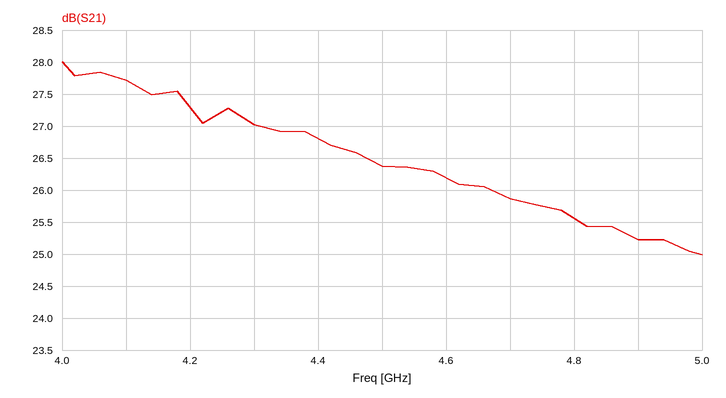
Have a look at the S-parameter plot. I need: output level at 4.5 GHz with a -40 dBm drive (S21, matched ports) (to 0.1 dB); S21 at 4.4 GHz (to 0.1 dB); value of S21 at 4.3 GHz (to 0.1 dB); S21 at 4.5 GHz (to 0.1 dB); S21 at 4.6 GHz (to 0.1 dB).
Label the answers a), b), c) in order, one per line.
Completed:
a) -13.6 dBm
b) 26.8 dB
c) 27.0 dB
d) 26.4 dB
e) 26.2 dB
